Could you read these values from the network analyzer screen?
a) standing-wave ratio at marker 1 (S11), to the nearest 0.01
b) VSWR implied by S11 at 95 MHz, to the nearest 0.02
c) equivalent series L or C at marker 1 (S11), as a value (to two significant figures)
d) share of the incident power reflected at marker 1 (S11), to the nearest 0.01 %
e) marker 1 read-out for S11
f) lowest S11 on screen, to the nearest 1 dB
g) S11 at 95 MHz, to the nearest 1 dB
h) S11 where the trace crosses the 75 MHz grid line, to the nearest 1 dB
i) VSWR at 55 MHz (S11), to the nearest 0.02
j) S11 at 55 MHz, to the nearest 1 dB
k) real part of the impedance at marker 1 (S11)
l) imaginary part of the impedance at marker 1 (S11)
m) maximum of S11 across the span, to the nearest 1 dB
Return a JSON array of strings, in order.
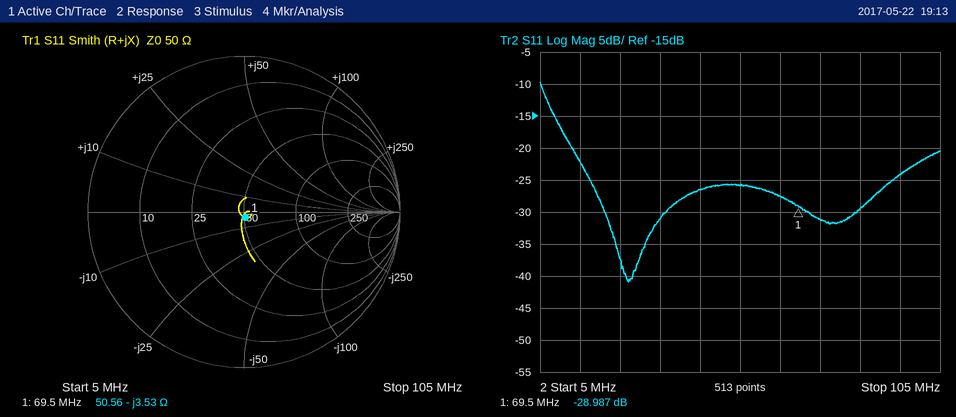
["1.07", "1.14", "650 pF", "0.13 %", "-28.987 dB", "-41 dB", "-24 dB", "-31 dB", "1.10", "-26 dB", "50.56 Ω", "-3.53 Ω", "-10 dB"]
